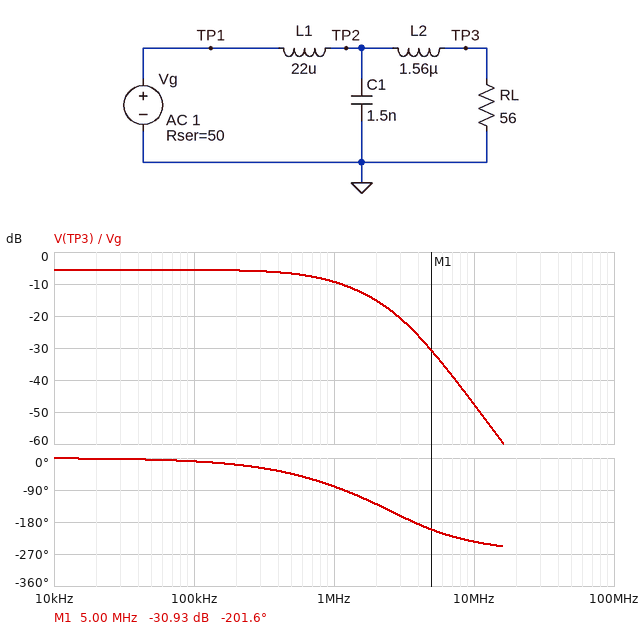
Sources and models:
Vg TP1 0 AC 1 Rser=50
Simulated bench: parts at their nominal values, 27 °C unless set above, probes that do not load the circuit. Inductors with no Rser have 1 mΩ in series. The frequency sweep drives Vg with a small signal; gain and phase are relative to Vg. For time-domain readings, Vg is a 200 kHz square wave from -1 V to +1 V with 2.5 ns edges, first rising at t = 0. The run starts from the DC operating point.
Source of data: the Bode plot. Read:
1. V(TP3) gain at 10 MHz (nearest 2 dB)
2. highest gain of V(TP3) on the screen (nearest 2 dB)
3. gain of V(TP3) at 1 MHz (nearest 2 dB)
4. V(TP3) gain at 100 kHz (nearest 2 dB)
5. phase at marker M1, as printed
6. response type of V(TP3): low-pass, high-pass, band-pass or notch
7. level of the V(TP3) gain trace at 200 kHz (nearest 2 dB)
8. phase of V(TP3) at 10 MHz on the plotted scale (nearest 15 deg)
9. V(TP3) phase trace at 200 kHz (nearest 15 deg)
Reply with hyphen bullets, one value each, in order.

- -48 dB
- -6 dB
- -10 dB
- -6 dB
- -201.6 deg
- low-pass
- -6 dB
- -240 deg
- -15 deg
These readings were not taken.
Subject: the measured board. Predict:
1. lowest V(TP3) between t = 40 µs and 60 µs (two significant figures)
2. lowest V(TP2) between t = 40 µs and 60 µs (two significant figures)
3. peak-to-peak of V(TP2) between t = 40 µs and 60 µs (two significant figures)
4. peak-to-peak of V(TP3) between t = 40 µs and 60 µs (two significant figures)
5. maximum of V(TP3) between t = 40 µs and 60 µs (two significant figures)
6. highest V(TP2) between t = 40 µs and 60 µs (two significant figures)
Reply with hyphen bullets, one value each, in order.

- -530 mV
- -530 mV
- 1.1 V
- 1.1 V
- 530 mV
- 530 mV
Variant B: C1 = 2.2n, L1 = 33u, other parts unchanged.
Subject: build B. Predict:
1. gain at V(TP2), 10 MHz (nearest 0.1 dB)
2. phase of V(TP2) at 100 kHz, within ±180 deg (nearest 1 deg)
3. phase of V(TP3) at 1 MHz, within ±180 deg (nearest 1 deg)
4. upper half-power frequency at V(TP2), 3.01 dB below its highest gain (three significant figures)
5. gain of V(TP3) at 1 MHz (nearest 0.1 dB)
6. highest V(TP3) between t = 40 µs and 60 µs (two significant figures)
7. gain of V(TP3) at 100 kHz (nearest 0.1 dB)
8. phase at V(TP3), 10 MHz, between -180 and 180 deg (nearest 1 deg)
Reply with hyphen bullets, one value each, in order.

- -48.6 dB
- -13 deg
- -105 deg
- 576 kHz
- -12.5 dB
- 530 mV
- -5.7 dB
- 123 deg
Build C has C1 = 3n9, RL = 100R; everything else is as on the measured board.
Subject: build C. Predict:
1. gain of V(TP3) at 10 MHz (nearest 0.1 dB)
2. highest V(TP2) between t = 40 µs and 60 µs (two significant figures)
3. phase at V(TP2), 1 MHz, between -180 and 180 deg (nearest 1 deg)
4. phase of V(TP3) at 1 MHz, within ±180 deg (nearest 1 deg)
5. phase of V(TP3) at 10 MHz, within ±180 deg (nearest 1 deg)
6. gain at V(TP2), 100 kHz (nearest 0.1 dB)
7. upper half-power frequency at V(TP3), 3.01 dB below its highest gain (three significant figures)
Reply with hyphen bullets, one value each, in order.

- -53.3 dB
- 810 mV
- -125 deg
- -130 deg
- 139 deg
- -3.5 dB
- 766 kHz
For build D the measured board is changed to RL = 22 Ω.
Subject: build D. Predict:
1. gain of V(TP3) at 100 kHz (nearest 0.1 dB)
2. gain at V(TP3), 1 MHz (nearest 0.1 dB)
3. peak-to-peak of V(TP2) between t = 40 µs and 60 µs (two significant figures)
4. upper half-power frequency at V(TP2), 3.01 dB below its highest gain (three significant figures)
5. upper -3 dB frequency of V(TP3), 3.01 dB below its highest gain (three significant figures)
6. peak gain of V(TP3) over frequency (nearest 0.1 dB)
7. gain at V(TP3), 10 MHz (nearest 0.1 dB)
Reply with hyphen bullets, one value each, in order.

- -10.5 dB
- -16.7 dB
- 610 mV
- 546 kHz
- 515 kHz
- -10.3 dB
- -54.5 dB
